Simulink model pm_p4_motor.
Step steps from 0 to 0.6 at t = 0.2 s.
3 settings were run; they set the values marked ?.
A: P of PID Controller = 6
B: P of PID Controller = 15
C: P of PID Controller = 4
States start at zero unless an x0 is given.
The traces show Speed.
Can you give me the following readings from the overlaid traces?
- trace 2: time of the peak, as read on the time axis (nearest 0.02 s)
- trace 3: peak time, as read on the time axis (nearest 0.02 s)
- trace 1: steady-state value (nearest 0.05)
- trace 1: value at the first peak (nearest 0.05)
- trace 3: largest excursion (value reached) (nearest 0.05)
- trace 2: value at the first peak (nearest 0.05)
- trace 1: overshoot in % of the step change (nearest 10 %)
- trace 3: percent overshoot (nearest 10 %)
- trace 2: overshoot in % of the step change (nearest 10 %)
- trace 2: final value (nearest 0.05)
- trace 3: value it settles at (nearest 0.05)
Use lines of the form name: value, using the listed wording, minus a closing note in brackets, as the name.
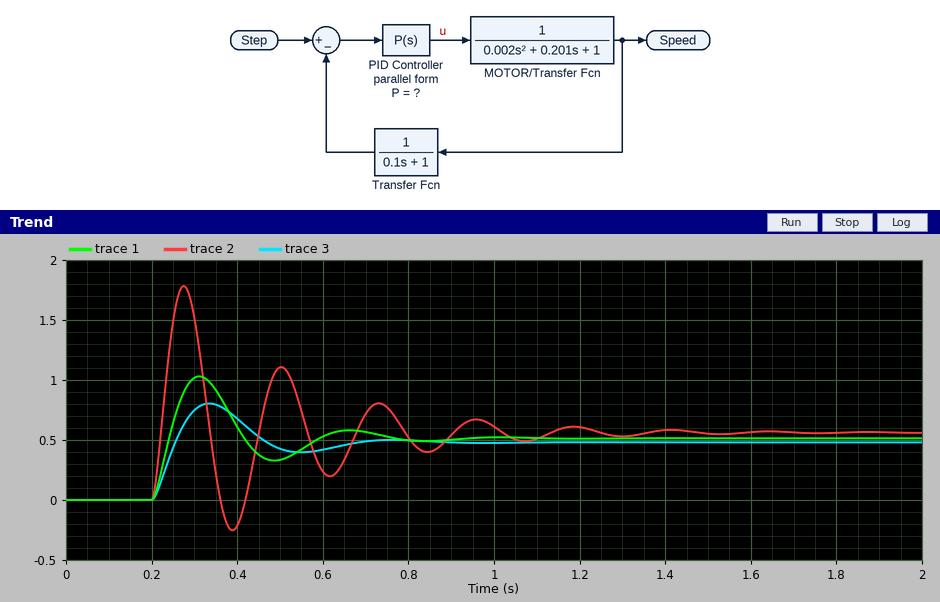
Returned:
trace 2: time of the peak, as read on the time axis: 0.28 s
trace 3: peak time, as read on the time axis: 0.34 s
trace 1: steady-state value: 0.50
trace 1: value at the first peak: 1.05
trace 3: largest excursion (value reached): 0.80
trace 2: value at the first peak: 1.80
trace 1: overshoot in % of the step change: 100 %
trace 3: percent overshoot: 70 %
trace 2: overshoot in % of the step change: 220 %
trace 2: final value: 0.55
trace 3: value it settles at: 0.50
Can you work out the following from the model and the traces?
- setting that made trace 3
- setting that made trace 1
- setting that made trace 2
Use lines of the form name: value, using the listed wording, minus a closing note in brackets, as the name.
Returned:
setting that made trace 3: C
setting that made trace 1: A
setting that made trace 2: B
